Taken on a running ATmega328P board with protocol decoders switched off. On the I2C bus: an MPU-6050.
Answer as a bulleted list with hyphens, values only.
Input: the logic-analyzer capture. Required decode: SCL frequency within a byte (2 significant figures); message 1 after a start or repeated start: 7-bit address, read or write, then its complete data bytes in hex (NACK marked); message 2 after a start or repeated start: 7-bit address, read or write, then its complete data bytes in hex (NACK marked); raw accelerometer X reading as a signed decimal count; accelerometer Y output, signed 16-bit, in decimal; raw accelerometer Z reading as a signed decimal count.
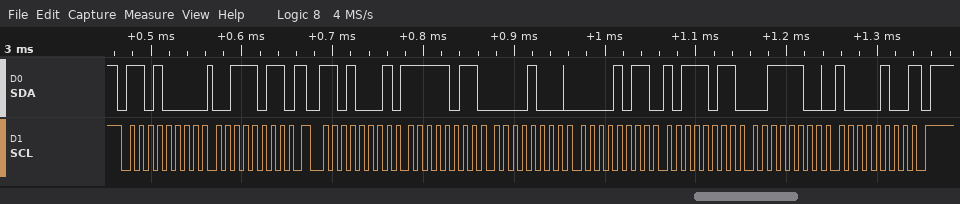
- 100 kHz
- 0x68 write: 3B
- 0x68 read: FB 08 0B BB 3C 84 NACK
- -1272
- 3003
- 15492
